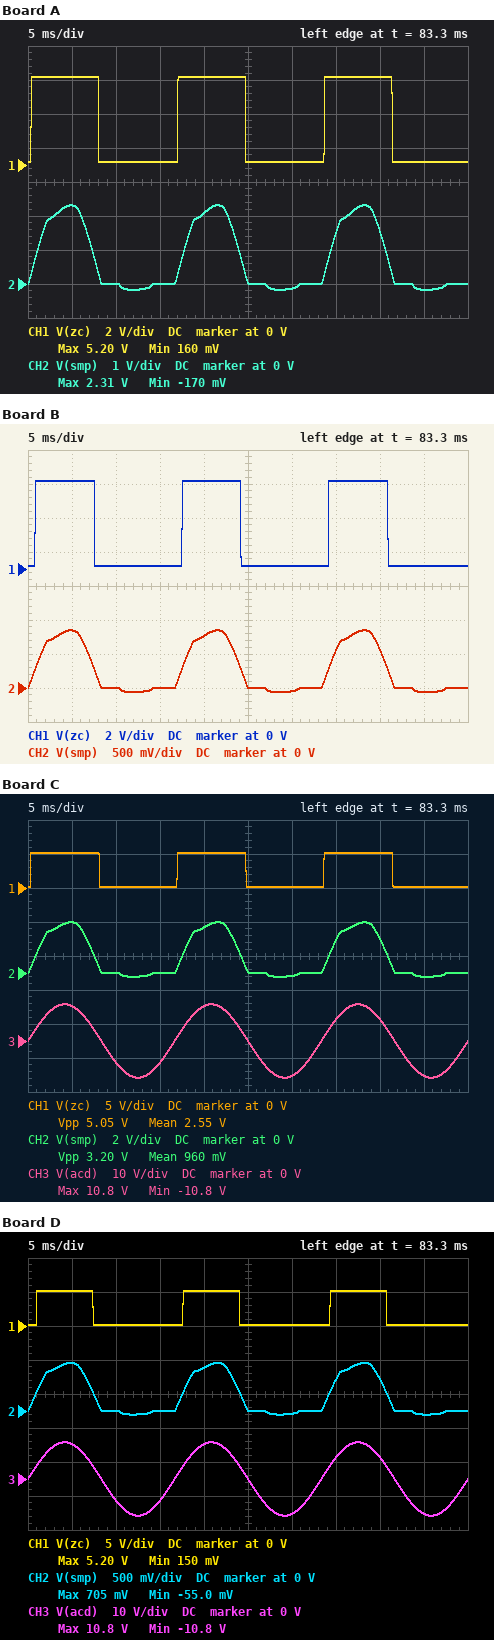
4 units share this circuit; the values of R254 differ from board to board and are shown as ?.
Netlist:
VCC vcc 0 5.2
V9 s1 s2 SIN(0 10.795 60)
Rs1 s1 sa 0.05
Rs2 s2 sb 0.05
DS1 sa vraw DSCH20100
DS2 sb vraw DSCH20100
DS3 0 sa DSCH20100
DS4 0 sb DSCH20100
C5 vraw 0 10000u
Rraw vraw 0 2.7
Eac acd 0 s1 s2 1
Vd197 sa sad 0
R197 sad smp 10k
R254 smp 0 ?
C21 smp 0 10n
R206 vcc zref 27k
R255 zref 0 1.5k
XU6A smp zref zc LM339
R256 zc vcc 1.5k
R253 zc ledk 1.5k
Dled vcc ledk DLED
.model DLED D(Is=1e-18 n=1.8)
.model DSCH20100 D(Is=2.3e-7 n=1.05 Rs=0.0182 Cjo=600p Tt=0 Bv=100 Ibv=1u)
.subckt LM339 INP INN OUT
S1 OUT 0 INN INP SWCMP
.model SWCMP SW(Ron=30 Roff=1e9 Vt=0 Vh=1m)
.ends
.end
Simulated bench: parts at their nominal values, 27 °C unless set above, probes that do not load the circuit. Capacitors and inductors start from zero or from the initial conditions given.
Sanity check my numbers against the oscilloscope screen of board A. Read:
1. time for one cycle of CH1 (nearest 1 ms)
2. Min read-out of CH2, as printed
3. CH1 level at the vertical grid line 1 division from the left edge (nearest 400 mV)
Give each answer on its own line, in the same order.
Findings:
17 ms
-170 mV
5.2 V
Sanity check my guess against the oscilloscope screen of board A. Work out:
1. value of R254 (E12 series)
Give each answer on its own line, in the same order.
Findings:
3.3 kΩ
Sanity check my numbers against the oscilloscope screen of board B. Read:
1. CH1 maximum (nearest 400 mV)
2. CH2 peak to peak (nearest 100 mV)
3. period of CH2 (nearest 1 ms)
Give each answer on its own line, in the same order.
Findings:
5.2 V
900 mV
17 ms
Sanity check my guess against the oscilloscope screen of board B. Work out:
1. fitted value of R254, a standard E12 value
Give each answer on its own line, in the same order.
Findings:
1 kΩ
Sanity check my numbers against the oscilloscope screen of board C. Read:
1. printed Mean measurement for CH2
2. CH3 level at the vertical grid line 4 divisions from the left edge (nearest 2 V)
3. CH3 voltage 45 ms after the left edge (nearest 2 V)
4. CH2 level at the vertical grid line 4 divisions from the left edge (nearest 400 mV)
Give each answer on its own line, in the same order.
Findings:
960 mV
10 V
-10 V
2.8 V
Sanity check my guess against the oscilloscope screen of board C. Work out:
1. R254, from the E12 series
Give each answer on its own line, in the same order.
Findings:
4.7 kΩ
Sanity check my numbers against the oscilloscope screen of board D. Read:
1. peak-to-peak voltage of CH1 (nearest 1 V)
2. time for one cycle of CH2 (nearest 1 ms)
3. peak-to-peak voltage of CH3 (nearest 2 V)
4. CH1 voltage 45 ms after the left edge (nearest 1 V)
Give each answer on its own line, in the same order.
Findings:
5 V
17 ms
22 V
0 V
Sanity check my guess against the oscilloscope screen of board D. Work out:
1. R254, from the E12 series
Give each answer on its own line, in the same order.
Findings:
820 Ω
